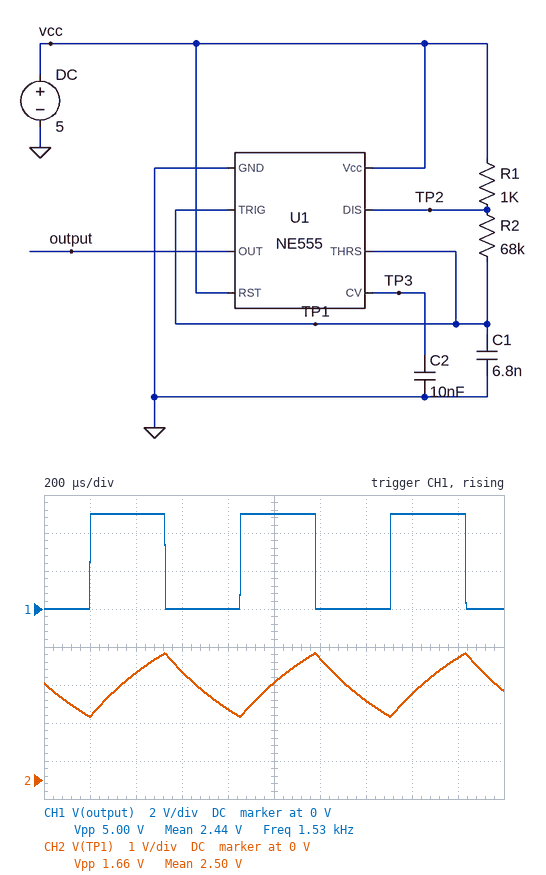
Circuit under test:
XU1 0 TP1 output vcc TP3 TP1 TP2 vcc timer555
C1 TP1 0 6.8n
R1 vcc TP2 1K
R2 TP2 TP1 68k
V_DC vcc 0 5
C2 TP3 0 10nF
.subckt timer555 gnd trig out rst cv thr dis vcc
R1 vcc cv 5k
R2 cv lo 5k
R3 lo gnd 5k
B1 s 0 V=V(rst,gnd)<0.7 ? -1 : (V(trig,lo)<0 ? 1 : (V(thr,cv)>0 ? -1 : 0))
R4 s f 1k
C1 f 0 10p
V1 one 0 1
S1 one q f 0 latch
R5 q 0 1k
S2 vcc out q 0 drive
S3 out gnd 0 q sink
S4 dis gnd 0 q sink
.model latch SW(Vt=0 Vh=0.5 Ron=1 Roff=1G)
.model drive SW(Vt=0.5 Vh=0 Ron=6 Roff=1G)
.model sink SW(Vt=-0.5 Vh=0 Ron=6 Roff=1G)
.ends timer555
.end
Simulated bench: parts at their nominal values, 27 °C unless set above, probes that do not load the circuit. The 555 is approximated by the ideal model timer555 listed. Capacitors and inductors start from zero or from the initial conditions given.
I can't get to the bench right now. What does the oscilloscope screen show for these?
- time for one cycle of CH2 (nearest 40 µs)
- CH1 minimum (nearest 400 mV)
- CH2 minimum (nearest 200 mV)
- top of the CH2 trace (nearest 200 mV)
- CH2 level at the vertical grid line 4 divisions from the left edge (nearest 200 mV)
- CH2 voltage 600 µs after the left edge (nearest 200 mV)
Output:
640 µs
0 V
1.6 V
3.4 V
1.8 V
2.8 V
